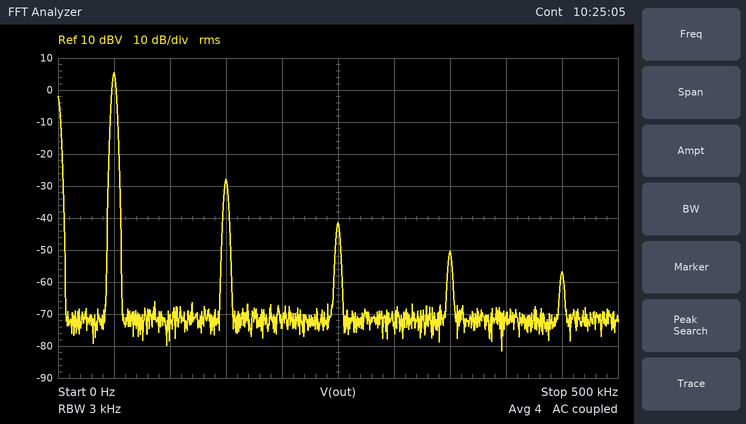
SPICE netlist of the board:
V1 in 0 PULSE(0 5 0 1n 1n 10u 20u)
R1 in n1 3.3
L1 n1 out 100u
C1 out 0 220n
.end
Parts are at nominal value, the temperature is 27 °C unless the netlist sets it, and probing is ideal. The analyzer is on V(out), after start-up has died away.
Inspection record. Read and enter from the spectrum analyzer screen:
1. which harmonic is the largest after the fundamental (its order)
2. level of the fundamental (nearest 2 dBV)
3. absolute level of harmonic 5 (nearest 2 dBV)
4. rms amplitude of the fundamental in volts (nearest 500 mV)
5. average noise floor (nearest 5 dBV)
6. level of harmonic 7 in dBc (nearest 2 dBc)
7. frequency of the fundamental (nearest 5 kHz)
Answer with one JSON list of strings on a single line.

["3", "6 dBV", "-42 dBV", "2.0 V", "-70 dBV", "-56 dBc", "50 kHz"]
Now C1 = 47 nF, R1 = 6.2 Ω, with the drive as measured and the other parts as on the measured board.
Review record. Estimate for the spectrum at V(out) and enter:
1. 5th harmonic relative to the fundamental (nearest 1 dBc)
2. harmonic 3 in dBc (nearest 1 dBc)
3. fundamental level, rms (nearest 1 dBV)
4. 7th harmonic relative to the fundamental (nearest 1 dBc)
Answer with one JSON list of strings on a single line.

["-40 dBc", "-25 dBc", "12 dBV", "-49 dBc"]
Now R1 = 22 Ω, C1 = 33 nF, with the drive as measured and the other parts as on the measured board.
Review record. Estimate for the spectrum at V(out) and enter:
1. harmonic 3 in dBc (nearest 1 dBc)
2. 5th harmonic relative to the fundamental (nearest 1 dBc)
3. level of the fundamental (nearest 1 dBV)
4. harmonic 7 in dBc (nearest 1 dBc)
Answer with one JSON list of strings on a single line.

["-19 dBc", "-34 dBc", "10 dBV", "-43 dBc"]
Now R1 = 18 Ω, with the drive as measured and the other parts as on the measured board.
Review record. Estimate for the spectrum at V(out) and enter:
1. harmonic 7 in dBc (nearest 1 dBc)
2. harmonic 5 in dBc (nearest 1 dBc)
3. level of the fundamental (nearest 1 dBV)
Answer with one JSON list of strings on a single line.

["-53 dBc", "-44 dBc", "2 dBV"]
